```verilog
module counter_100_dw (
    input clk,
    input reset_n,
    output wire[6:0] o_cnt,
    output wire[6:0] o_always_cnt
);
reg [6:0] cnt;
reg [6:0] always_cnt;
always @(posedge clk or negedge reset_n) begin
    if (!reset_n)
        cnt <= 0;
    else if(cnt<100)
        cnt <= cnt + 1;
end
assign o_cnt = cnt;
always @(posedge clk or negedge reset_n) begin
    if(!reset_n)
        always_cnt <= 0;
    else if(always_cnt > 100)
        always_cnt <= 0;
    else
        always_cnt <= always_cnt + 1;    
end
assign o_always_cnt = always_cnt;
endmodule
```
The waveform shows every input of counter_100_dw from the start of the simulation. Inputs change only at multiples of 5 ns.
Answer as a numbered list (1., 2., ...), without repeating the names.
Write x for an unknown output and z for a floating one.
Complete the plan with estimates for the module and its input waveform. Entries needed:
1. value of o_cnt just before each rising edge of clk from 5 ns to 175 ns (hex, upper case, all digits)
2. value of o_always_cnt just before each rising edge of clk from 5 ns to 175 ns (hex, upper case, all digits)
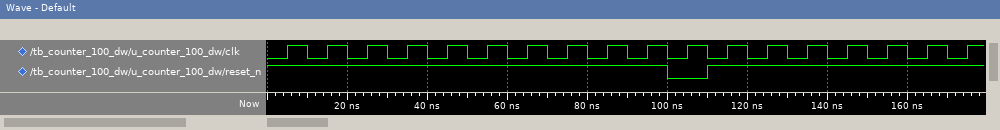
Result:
1. x, x, x, x, x, x, x, x, x, x, 00, 00, 01, 02, 03, 04, 05, 06
2. x, x, x, x, x, x, x, x, x, x, 00, 00, 01, 02, 03, 04, 05, 06
